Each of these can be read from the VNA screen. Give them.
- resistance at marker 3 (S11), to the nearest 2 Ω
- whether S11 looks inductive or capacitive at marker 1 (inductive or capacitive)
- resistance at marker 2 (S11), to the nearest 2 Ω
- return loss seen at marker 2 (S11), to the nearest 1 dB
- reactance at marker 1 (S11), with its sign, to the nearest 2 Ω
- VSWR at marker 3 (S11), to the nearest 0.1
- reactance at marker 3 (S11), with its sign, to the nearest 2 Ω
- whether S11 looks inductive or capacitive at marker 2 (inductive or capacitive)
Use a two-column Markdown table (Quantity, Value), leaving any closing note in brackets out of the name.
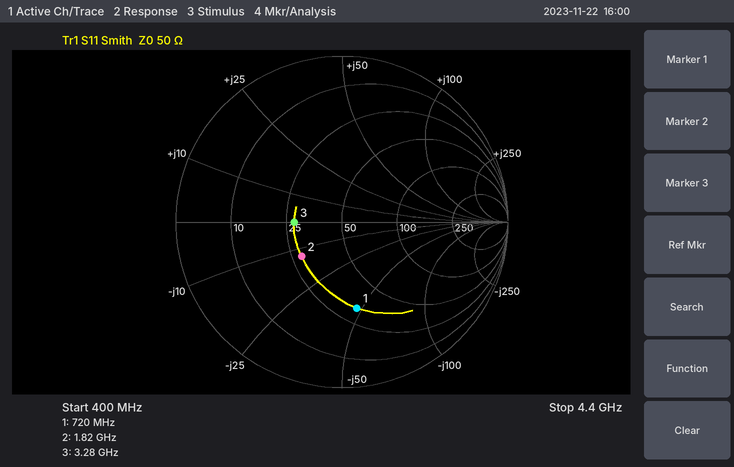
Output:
| Quantity | Value |
|---|---|
| resistance at marker 3 (S11), to the nearest 2 Ω | 28 Ω |
| whether S11 looks inductive or capacitive at marker 1 | capacitive |
| resistance at marker 2 (S11), to the nearest 2 Ω | 28 Ω |
| return loss seen at marker 2 (S11), to the nearest 1 dB | 10 dB |
| reactance at marker 1 (S11), with its sign, to the nearest 2 Ω | -48 Ω |
| VSWR at marker 3 (S11), to the nearest 0.1 | 1.8 |
| reactance at marker 3 (S11), with its sign, to the nearest 2 Ω | 0 Ω |
| whether S11 looks inductive or capacitive at marker 2 | capacitive |
